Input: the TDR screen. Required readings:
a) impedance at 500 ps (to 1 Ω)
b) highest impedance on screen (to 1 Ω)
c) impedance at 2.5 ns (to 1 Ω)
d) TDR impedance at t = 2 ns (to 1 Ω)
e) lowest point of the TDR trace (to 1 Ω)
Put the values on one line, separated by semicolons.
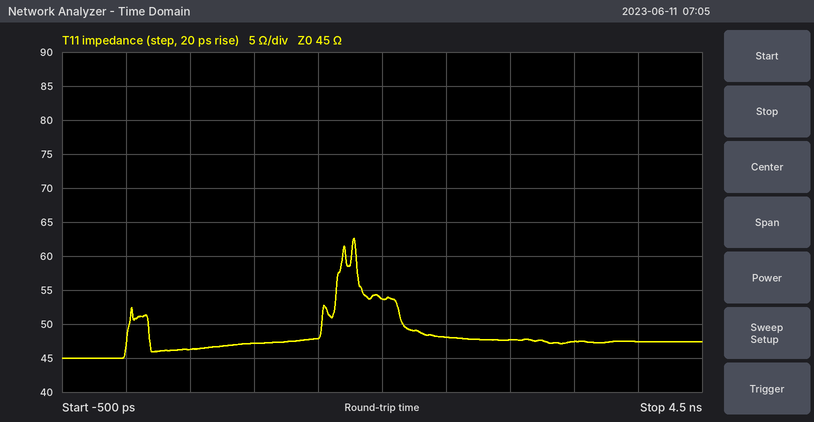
46 Ω; 63 Ω; 48 Ω; 54 Ω; 45 Ω
